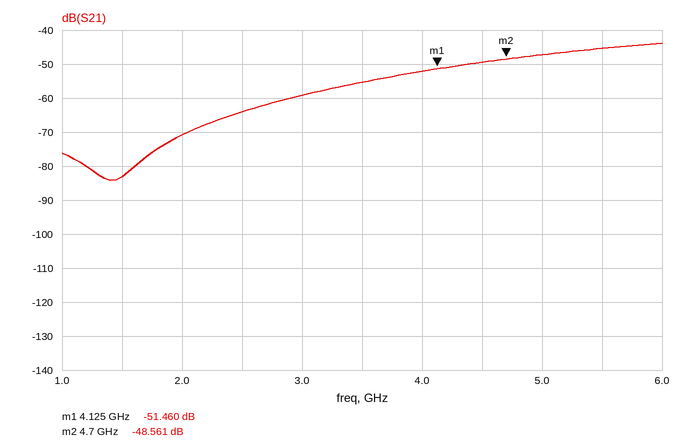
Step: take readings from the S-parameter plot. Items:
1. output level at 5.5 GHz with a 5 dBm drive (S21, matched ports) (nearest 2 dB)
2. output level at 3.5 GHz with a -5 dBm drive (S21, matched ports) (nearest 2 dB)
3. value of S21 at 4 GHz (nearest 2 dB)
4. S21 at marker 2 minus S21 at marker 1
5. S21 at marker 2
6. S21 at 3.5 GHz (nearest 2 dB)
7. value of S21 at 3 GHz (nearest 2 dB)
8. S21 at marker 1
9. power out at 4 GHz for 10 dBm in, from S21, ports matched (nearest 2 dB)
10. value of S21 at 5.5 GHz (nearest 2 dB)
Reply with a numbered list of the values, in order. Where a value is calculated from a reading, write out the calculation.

1. 5 dBm + (-46 dB) = -40 dBm
2. -5 dBm + (-56 dB) = -60 dBm
3. -52 dB
4. -48.561 − (-51.46) = 2.899 dB
5. -48.561 dB
6. -56 dB
7. -60 dB
8. -51.460 dB
9. 10 dBm + (-52 dB) = -42 dBm
10. -46 dB
